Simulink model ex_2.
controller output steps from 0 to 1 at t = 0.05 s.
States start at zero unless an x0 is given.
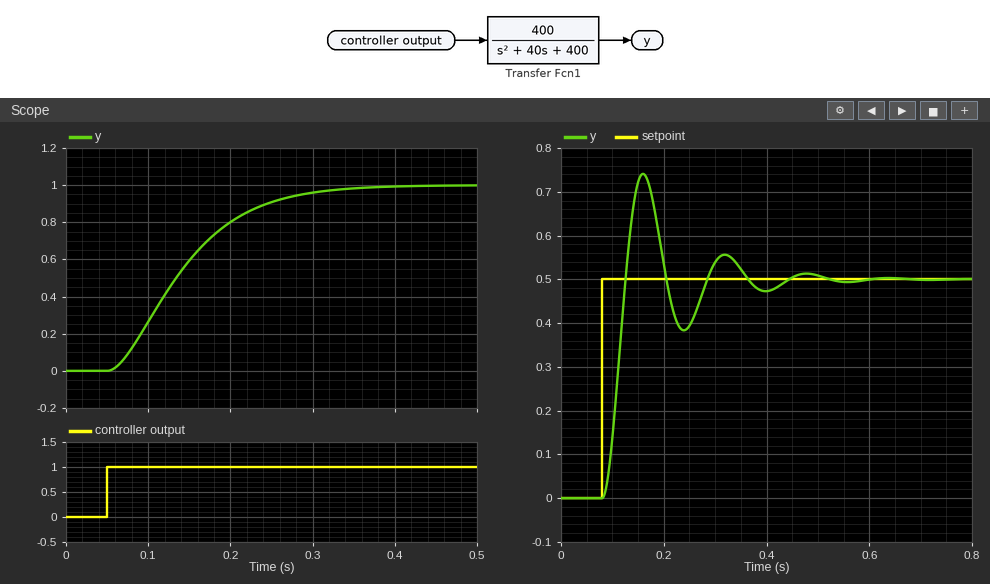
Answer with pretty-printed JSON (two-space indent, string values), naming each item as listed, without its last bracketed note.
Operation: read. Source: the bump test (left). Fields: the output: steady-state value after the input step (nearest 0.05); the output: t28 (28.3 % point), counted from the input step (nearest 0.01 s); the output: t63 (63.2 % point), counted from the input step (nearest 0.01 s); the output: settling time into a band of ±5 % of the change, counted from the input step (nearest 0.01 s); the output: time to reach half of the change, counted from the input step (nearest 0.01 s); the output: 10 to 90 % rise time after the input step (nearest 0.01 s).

{
  "the output: steady-state value after the input step": "1.00",
  "the output: t28 (28.3 % point), counted from the input step": "0.05 s",
  "the output: t63 (63.2 % point), counted from the input step": "0.11 s",
  "the output: settling time into a band of ±5 % of the change, counted from the input step": "0.24 s",
  "the output: time to reach half of the change, counted from the input step": "0.08 s",
  "the output: 10 to 90 % rise time after the input step": "0.17 s"
}
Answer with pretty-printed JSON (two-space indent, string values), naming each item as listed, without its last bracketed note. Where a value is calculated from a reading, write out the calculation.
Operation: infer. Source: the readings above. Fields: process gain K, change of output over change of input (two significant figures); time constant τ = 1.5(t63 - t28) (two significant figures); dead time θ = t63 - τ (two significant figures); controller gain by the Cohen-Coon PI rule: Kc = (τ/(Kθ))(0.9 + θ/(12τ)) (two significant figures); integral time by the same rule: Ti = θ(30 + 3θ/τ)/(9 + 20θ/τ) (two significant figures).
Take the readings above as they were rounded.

{
  "process gain K, change of output over change of input": "(1 - 0) / 1 = 1.0",
  "time constant τ = 1.5(t63 - t28)": "1.5 × (0.11 - 0.05) = 0.090 s",
  "dead time θ = t63 - τ": "0.11 - 0.09 = 0.020 s",
  "controller gain by the Cohen-Coon PI rule: Kc = (τ/(Kθ))(0.9 + θ/(12τ))": "0.09 / (1 × 0.02) × (0.9 + 0.02 / (12 × 0.09)) = 4.1",
  "integral time by the same rule: Ti = θ(30 + 3θ/τ)/(9 + 20θ/τ)": "0.02 × (30 + 3 × 0.02 / 0.09) / (9 + 20 × 0.02 / 0.09) = 0.046 s"
}
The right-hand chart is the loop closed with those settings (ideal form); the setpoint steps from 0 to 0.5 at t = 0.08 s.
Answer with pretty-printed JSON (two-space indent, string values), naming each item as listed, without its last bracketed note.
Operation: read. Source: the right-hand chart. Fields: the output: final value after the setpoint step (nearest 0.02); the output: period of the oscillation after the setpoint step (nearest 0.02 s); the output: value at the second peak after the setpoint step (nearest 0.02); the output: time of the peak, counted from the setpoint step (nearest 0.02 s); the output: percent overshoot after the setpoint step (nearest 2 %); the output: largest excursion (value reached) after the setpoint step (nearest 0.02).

{
  "the output: final value after the setpoint step": "0.50",
  "the output: period of the oscillation after the setpoint step": "0.16 s",
  "the output: value at the second peak after the setpoint step": "0.56",
  "the output: time of the peak, counted from the setpoint step": "0.08 s",
  "the output: percent overshoot after the setpoint step": "48 %",
  "the output: largest excursion (value reached) after the setpoint step": "0.74"
}
